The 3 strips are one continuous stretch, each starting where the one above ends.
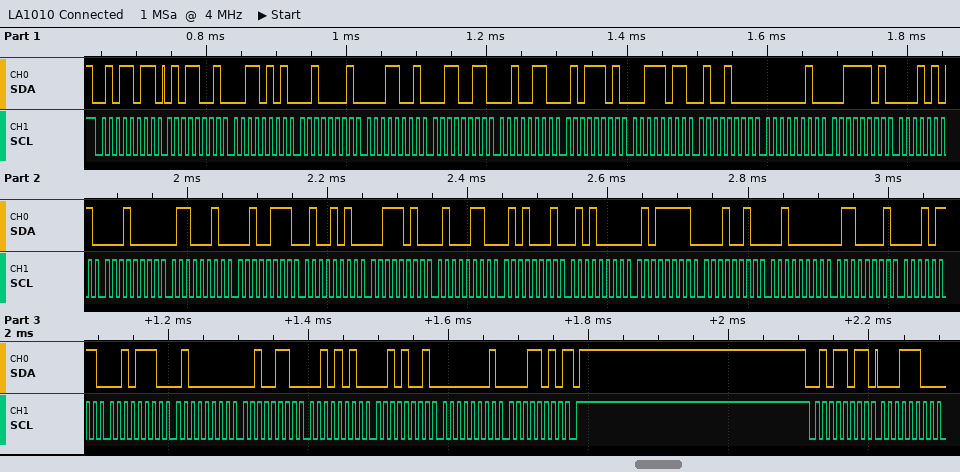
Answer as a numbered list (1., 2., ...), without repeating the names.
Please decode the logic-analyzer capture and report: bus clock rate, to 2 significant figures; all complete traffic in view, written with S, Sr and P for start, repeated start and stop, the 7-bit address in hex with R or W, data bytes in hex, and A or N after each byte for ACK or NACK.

1. 100 kHz
2. S 2DR A 59 A 35 A 21 A 19 A 33 A 26 A 5D A 3B A 48 A 02 A 3D A 15 A 10 A 62 A 27 A 4A A 3A A 46 A 51 A 50 A 5F A 12 A 20 A 61 A 17 A 2E A 40 A 26 A 2A A 29 A 01 A 1A N P S 2DR A 1C A
